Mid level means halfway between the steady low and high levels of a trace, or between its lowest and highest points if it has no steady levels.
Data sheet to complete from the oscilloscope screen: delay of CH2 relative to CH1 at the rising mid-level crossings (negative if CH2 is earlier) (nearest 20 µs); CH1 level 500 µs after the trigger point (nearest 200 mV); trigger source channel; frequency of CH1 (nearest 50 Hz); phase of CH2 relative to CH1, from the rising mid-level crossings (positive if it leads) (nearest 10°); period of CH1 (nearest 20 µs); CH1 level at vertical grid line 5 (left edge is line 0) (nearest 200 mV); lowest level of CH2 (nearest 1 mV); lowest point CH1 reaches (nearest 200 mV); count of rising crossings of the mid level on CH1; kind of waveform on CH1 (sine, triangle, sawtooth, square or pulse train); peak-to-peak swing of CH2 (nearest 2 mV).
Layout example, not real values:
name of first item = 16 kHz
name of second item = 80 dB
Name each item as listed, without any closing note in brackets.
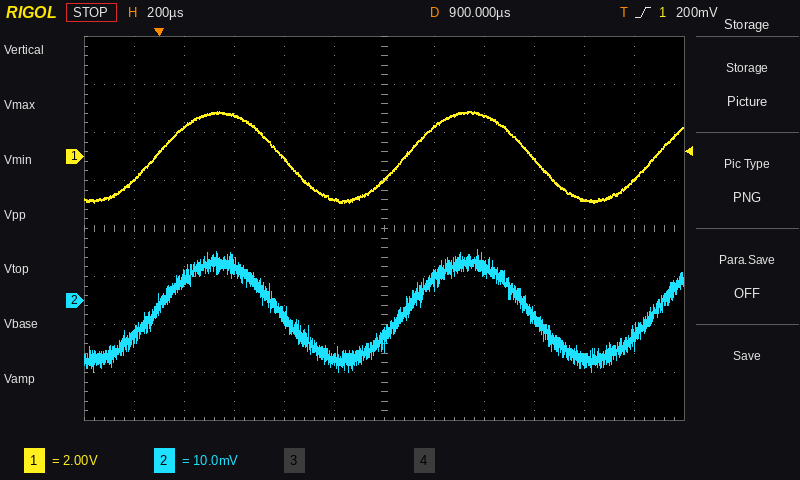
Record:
delay of CH2 relative to CH1 at the rising mid-level crossings (negative if CH2 is earlier) = 0 µs
CH1 level 500 µs after the trigger point = 0.0 V
trigger source channel = CH1
frequency of CH1 = 1.00 kHz
phase of CH2 relative to CH1, from the rising mid-level crossings (positive if it leads) = 0°
period of CH1 = 1.00 ms
CH1 level at vertical grid line 5 (left edge is line 0) = -1.8 V
lowest level of CH2 = -15 mV
lowest point CH1 reaches = -2.0 V
count of rising crossings of the mid level on CH1 = 3
kind of waveform on CH1 = sine
peak-to-peak swing of CH2 = 26 mV
